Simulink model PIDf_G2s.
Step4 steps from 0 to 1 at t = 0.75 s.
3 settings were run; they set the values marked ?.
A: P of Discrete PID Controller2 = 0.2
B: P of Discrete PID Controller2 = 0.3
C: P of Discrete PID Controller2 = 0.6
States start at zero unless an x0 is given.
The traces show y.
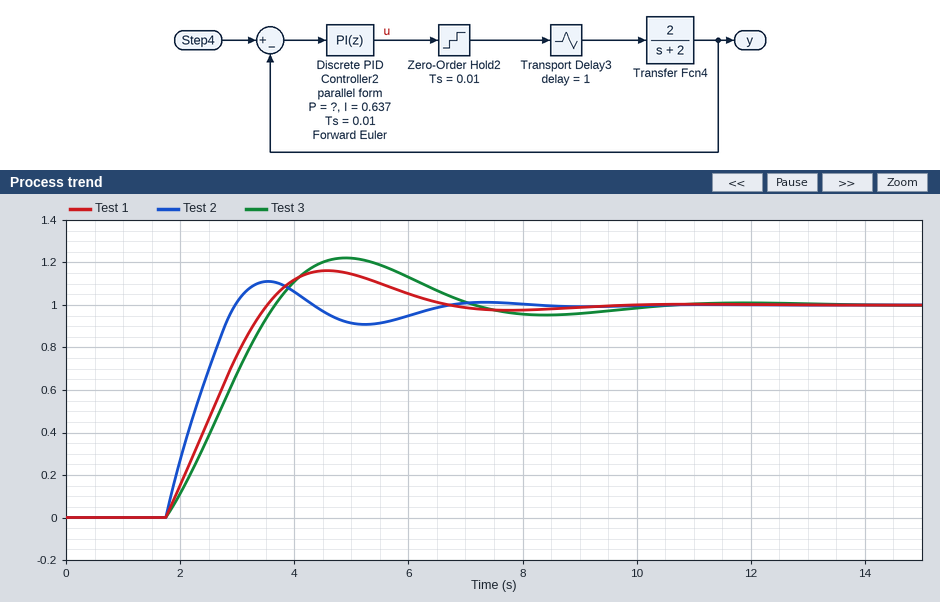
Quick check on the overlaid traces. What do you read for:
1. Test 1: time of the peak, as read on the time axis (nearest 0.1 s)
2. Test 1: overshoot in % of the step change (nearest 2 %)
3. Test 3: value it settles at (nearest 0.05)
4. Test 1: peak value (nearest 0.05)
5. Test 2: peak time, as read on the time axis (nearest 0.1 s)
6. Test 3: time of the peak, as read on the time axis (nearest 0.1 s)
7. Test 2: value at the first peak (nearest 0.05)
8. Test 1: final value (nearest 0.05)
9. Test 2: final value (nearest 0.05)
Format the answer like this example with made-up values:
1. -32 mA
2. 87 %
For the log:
1. 4.6 s
2. 16 %
3. 1.00
4. 1.15
5. 3.5 s
6. 4.9 s
7. 1.10
8. 1.00
9. 1.00
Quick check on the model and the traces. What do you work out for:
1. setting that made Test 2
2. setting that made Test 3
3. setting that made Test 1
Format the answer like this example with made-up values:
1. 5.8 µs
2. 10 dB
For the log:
1. C
2. A
3. B
